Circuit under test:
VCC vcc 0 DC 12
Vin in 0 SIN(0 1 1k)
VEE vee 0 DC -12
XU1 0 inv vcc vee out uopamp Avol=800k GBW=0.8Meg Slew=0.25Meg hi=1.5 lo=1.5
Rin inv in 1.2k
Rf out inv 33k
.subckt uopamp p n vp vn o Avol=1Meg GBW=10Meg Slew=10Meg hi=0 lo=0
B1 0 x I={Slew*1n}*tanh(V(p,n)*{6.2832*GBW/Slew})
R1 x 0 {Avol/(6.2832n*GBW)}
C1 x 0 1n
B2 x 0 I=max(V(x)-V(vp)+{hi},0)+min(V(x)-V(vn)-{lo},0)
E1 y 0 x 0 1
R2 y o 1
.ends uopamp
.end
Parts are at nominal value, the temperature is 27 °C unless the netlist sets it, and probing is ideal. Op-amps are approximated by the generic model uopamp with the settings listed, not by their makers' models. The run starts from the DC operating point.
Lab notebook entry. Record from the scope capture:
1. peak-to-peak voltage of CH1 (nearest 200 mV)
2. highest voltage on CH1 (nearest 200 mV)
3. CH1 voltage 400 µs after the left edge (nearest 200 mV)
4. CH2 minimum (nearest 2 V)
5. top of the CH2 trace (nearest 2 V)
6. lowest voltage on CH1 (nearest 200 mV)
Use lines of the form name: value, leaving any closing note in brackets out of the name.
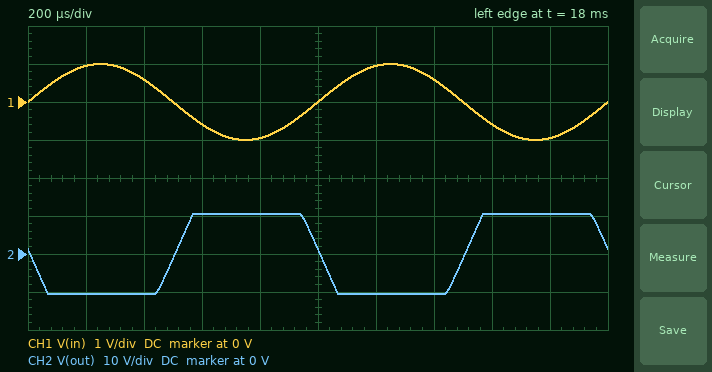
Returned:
peak-to-peak voltage of CH1: 2.0 V
highest voltage on CH1: 1.0 V
CH1 voltage 400 µs after the left edge: 600 mV
CH2 minimum: -10 V
top of the CH2 trace: 10 V
lowest voltage on CH1: -1.0 V
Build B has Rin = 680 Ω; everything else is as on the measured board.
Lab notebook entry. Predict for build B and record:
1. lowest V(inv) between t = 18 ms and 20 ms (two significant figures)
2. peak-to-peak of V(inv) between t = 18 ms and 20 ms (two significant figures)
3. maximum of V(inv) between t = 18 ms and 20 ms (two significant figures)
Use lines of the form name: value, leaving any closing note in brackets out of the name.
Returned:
lowest V(inv) between t = 18 ms and 20 ms: -770 mV
peak-to-peak of V(inv) between t = 18 ms and 20 ms: 1.5 V
maximum of V(inv) between t = 18 ms and 20 ms: 770 mV
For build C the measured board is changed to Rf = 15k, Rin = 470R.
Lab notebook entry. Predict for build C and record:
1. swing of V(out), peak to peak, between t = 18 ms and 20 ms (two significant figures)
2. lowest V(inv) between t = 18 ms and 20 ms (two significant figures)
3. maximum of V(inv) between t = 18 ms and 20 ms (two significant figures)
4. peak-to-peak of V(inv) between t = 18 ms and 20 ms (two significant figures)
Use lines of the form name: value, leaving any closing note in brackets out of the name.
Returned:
swing of V(out), peak to peak, between t = 18 ms and 20 ms: 21 V
lowest V(inv) between t = 18 ms and 20 ms: -650 mV
maximum of V(inv) between t = 18 ms and 20 ms: 650 mV
peak-to-peak of V(inv) between t = 18 ms and 20 ms: 1.3 V
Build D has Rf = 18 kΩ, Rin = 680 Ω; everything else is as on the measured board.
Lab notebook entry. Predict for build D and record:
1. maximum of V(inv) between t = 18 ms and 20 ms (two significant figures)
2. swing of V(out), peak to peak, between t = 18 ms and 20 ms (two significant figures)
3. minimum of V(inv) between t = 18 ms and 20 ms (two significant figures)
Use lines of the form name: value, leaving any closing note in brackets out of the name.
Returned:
maximum of V(inv) between t = 18 ms and 20 ms: 580 mV
swing of V(out), peak to peak, between t = 18 ms and 20 ms: 21 V
minimum of V(inv) between t = 18 ms and 20 ms: -580 mV
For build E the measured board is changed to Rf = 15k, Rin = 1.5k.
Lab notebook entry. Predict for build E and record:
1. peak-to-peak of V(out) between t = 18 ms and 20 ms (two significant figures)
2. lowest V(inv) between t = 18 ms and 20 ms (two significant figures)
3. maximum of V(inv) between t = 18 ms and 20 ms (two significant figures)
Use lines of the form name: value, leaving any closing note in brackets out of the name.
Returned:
peak-to-peak of V(out) between t = 18 ms and 20 ms: 20 V
lowest V(inv) between t = 18 ms and 20 ms: -13 mV
maximum of V(inv) between t = 18 ms and 20 ms: 13 mV
